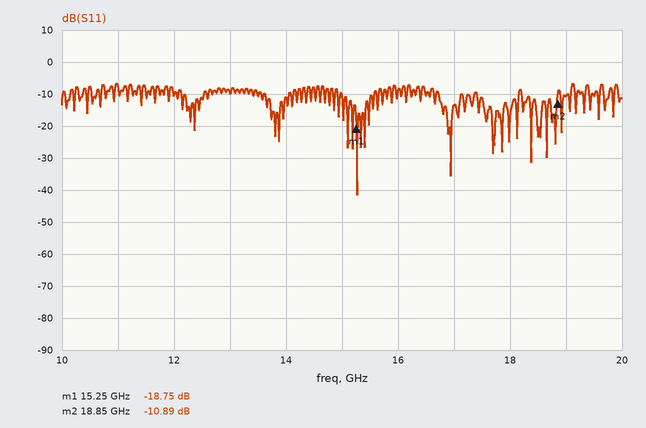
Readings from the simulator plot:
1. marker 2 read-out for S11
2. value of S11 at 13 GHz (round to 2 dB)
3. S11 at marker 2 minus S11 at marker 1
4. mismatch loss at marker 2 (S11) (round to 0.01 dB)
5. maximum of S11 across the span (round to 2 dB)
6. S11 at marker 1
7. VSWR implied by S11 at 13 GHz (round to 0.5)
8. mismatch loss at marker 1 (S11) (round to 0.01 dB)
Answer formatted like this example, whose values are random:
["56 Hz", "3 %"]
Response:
["-10.89 dB", "-10 dB", "7.86 dB", "0.37 dB", "-6 dB", "-18.75 dB", "2.0", "0.06 dB"]
